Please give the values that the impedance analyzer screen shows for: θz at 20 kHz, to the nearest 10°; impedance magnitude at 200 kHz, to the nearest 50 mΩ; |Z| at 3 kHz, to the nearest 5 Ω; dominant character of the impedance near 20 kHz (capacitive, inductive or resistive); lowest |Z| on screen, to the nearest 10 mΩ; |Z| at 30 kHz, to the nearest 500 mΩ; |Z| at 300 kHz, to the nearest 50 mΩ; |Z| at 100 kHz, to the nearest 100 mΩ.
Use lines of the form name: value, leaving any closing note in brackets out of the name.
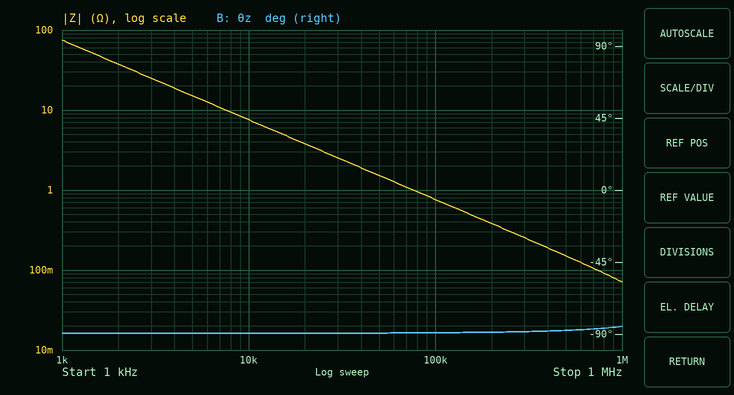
θz at 20 kHz, to the nearest 10°: -90°
impedance magnitude at 200 kHz, to the nearest 50 mΩ: 400 mΩ
|Z| at 3 kHz, to the nearest 5 Ω: 25 Ω
dominant character of the impedance near 20 kHz: capacitive
lowest |Z| on screen, to the nearest 10 mΩ: 70 mΩ
|Z| at 30 kHz, to the nearest 500 mΩ: 2.5 Ω
|Z| at 300 kHz, to the nearest 50 mΩ: 250 mΩ
|Z| at 100 kHz, to the nearest 100 mΩ: 800 mΩ
